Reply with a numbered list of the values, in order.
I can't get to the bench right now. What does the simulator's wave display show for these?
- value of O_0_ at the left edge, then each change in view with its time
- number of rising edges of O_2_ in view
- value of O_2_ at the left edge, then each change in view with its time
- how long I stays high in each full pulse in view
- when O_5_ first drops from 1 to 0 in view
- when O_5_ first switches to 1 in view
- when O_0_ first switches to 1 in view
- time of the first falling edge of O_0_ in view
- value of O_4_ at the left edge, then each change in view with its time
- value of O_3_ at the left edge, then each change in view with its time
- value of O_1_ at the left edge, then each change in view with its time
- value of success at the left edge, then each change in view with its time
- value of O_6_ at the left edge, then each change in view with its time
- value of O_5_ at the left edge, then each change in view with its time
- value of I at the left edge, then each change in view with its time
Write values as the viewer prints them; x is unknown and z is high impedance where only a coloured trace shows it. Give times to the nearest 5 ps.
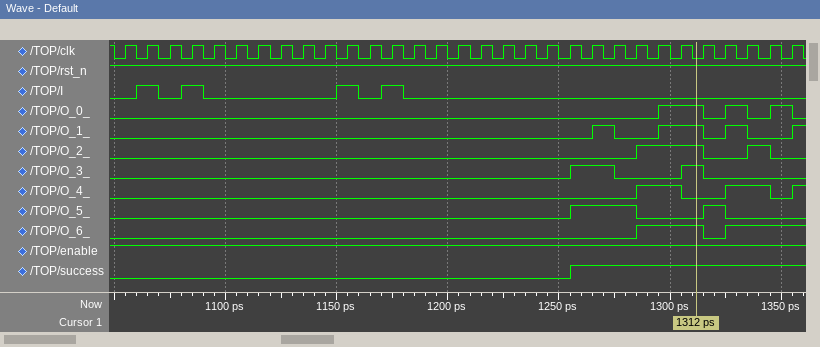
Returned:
1. 0, 1 at 1295 ps, 0 at 1315 ps, 1 at 1325 ps, 0 at 1335 ps, 1 at 1345 ps, 0 at 1355 ps
2. 2
3. 0, 1 at 1285 ps, 0 at 1315 ps, 1 at 1335 ps, 0 at 1345 ps
4. 10 ps, 10 ps, 10 ps, 10 ps
5. 1285 ps
6. 1255 ps
7. 1295 ps
8. 1315 ps
9. 0, 1 at 1285 ps, 0 at 1305 ps, 1 at 1325 ps, 0 at 1345 ps, 1 at 1355 ps
10. 0, 1 at 1255 ps, 0 at 1275 ps, 1 at 1305 ps, 0 at 1315 ps
11. 0, 1 at 1265 ps, 0 at 1275 ps, 1 at 1295 ps, 0 at 1315 ps, 1 at 1325 ps, 0 at 1335 ps, 1 at 1355 ps
12. 0, 1 at 1255 ps
13. 0, 1 at 1285 ps, 0 at 1315 ps, 1 at 1325 ps
14. 0, 1 at 1255 ps, 0 at 1285 ps, 1 at 1315 ps, 0 at 1325 ps
15. 0, 1 at 1060 ps, 0 at 1070 ps, 1 at 1080 ps, 0 at 1090 ps, 1 at 1150 ps, 0 at 1160 ps, 1 at 1170 ps, 0 at 1180 ps
